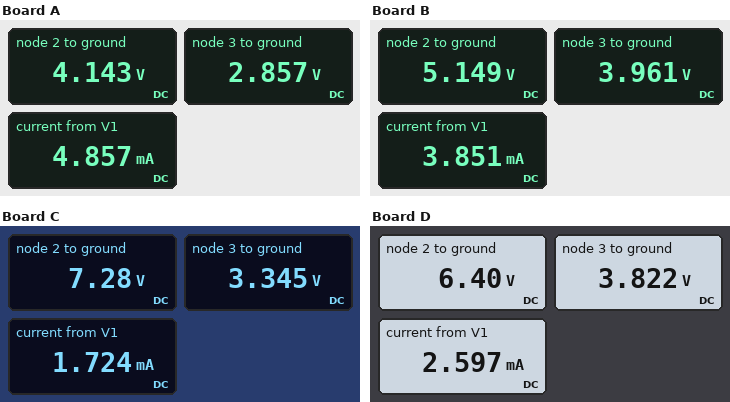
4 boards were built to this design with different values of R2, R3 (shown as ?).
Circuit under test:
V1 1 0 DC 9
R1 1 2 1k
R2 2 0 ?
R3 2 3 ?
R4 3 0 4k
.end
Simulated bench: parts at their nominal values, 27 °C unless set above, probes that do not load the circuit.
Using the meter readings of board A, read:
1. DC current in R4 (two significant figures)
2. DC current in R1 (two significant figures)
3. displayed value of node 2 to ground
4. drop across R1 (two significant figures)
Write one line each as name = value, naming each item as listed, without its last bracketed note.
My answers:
DC current in R4 = 710 µA
DC current in R1 = 4.9 mA
displayed value of node 2 to ground = 4.143 V
drop across R1 = 4.9 V
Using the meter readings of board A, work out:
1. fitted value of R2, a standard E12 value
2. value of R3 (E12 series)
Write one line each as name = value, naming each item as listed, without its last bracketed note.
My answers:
fitted value of R2, a standard E12 value = 1 kΩ
value of R3 = 1.8 kΩ
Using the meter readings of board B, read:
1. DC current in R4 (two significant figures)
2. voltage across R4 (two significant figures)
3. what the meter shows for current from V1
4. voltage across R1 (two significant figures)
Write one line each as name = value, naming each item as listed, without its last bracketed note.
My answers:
DC current in R4 = 990 µA
voltage across R4 = 4.0 V
what the meter shows for current from V1 = 3.851 mA
voltage across R1 = 3.9 V
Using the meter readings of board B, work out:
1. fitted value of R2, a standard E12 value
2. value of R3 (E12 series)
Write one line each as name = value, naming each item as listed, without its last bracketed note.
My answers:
fitted value of R2, a standard E12 value = 1.8 kΩ
value of R3 = 1.2 kΩ
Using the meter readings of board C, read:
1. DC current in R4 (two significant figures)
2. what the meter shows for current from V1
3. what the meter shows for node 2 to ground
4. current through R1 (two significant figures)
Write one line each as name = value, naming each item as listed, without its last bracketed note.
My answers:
DC current in R4 = 840 µA
what the meter shows for current from V1 = 1.724 mA
what the meter shows for node 2 to ground = 7.28 V
current through R1 = 1.7 mA
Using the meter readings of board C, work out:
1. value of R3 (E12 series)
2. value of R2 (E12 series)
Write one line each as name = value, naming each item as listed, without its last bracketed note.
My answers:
value of R3 = 4.7 kΩ
value of R2 = 8.2 kΩ
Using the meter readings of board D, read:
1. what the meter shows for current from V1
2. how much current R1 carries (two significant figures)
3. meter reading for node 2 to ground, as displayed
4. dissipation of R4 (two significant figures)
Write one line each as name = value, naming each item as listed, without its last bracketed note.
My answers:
what the meter shows for current from V1 = 2.597 mA
how much current R1 carries = 2.6 mA
meter reading for node 2 to ground, as displayed = 6.40 V
dissipation of R4 = 3.7 mW
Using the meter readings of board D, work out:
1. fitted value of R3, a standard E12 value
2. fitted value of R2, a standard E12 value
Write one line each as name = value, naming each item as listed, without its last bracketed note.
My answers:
fitted value of R3, a standard E12 value = 2.7 kΩ
fitted value of R2, a standard E12 value = 3.9 kΩ
